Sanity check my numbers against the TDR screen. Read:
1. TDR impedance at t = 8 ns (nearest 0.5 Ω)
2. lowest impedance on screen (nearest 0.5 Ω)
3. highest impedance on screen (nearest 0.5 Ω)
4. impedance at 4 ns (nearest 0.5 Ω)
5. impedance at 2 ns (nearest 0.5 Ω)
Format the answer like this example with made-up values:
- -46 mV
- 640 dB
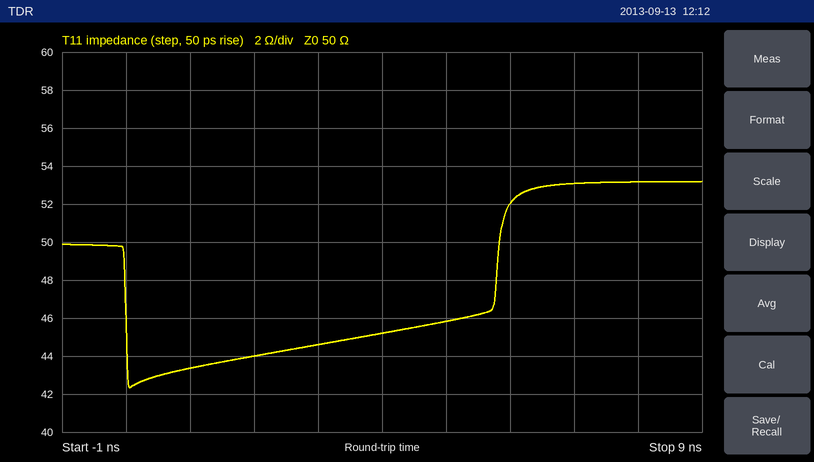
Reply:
- 53.0 Ω
- 42.5 Ω
- 53.0 Ω
- 45.0 Ω
- 44.0 Ω
